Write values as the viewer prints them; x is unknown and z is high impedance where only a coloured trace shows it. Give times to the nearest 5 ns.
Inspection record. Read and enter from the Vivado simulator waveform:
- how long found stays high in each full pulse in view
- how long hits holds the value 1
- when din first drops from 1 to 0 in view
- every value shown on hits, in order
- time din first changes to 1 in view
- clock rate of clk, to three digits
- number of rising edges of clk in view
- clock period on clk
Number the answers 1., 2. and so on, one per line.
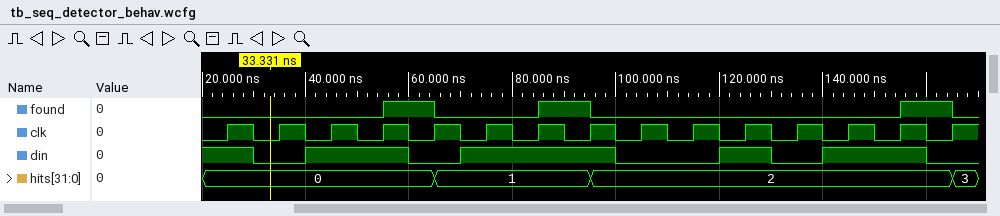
1. 10 ns, 10 ns, 10 ns
2. 30 ns
3. 30 ns
4. 0, 1, 2, 3
5. 40 ns
6. 100 MHz
7. 15
8. 10 ns
